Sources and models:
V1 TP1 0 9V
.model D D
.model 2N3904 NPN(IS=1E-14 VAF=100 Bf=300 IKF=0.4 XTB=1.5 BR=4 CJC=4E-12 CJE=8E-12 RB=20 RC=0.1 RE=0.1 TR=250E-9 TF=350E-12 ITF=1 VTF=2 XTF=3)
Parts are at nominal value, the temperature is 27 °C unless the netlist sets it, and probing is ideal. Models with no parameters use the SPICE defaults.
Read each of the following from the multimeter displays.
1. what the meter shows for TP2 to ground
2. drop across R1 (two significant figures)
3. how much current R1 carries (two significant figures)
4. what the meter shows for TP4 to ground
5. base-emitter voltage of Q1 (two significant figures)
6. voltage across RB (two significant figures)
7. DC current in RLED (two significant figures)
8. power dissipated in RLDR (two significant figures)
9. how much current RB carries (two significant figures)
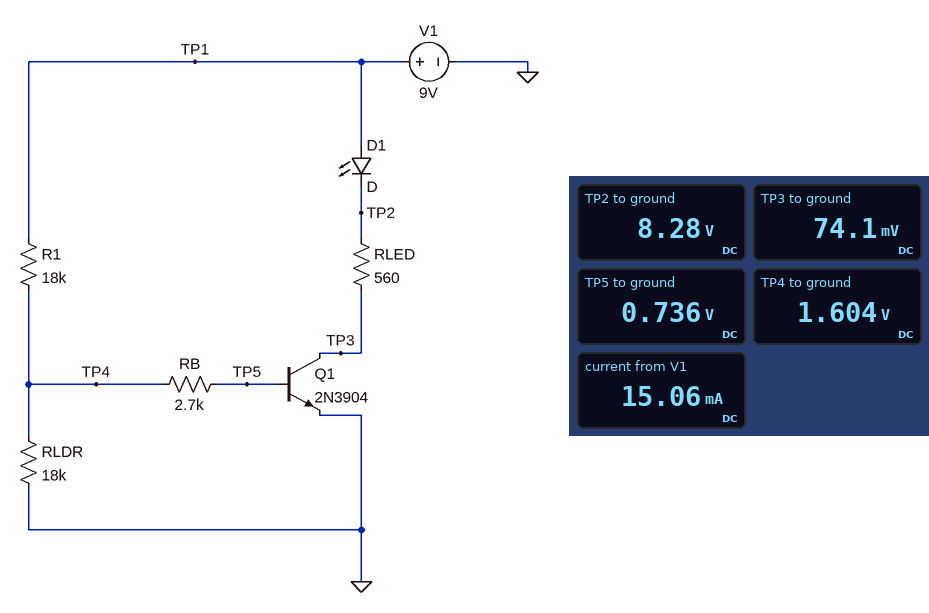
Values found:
8.28 V
7.4 V
410 µA
1.604 V
740 mV
870 mV
15 mA
140 µW
320 µA
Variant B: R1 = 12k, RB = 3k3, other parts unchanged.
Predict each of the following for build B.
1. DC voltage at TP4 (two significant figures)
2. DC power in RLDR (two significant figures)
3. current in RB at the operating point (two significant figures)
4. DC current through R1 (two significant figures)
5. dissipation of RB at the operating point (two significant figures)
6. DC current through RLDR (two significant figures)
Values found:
2.2 V
270 µW
440 µA
570 µA
650 µW
120 µA
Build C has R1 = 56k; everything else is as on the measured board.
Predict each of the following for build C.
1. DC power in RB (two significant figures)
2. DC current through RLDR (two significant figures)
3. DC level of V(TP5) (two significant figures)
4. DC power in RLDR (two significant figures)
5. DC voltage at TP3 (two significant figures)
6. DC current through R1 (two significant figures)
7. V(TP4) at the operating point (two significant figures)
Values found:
22 µW
54 µA
730 mV
52 µW
120 mV
140 µA
970 mV
